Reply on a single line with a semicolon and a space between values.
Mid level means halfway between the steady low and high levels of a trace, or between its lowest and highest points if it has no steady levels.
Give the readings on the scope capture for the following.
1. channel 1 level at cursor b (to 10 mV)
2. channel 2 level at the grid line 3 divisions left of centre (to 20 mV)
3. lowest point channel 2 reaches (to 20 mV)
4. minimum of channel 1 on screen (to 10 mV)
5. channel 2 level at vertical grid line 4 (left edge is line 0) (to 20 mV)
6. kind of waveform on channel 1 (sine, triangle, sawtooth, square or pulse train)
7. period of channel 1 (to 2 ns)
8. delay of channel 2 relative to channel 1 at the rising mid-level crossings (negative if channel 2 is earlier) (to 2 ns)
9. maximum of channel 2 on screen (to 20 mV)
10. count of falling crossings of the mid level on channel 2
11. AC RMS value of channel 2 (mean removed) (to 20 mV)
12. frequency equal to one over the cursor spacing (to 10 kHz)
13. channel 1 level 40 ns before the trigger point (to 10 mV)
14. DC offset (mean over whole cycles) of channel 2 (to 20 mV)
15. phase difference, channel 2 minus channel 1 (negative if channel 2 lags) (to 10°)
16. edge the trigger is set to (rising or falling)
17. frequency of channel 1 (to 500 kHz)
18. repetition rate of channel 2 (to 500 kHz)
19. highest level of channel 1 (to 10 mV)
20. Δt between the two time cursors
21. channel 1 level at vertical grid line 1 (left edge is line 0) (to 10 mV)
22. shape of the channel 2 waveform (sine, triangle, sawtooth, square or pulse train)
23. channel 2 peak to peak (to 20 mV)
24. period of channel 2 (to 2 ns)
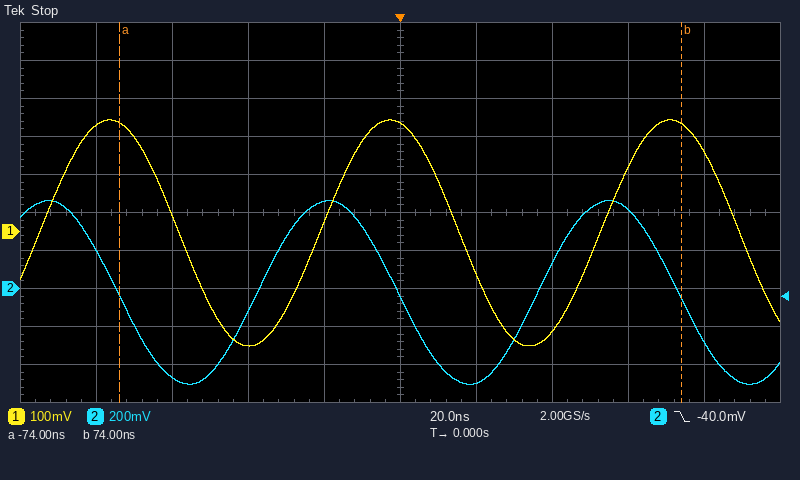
280 mV; -460 mV; -500 mV; -300 mV; 460 mV; sine; 74 ns; -16 ns; 460 mV; 3; 340 mV; 6.76 MHz; -300 mV; -20 mV; +80°; falling; 13.5 MHz; 13.5 MHz; 290 mV; 148 ns; 280 mV; sine; 960 mV; 74 ns
